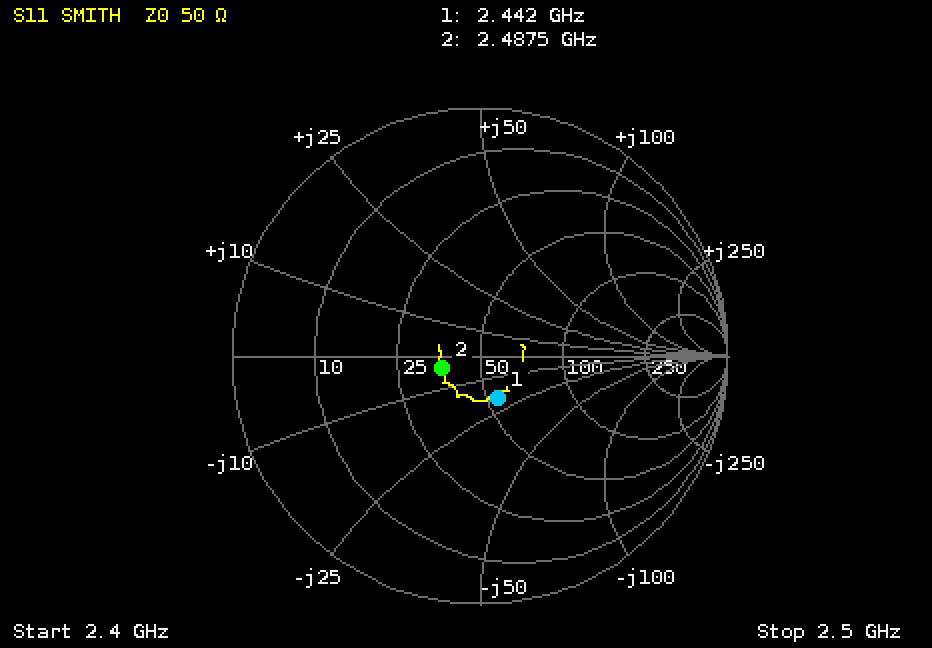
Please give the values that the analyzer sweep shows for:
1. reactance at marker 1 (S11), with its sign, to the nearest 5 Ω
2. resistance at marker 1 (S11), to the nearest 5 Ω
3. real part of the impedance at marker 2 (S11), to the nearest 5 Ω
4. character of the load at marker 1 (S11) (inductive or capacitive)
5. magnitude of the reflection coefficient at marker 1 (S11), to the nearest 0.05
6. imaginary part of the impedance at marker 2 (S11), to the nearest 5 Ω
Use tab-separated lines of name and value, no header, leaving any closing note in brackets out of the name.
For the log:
reactance at marker 1 (S11), with its sign, to the nearest 5 Ω	-20 Ω
resistance at marker 1 (S11), to the nearest 5 Ω	55 Ω
real part of the impedance at marker 2 (S11), to the nearest 5 Ω	35 Ω
character of the load at marker 1 (S11)	capacitive
magnitude of the reflection coefficient at marker 1 (S11), to the nearest 0.05	0.20
imaginary part of the impedance at marker 2 (S11), to the nearest 5 Ω	-5 Ω
